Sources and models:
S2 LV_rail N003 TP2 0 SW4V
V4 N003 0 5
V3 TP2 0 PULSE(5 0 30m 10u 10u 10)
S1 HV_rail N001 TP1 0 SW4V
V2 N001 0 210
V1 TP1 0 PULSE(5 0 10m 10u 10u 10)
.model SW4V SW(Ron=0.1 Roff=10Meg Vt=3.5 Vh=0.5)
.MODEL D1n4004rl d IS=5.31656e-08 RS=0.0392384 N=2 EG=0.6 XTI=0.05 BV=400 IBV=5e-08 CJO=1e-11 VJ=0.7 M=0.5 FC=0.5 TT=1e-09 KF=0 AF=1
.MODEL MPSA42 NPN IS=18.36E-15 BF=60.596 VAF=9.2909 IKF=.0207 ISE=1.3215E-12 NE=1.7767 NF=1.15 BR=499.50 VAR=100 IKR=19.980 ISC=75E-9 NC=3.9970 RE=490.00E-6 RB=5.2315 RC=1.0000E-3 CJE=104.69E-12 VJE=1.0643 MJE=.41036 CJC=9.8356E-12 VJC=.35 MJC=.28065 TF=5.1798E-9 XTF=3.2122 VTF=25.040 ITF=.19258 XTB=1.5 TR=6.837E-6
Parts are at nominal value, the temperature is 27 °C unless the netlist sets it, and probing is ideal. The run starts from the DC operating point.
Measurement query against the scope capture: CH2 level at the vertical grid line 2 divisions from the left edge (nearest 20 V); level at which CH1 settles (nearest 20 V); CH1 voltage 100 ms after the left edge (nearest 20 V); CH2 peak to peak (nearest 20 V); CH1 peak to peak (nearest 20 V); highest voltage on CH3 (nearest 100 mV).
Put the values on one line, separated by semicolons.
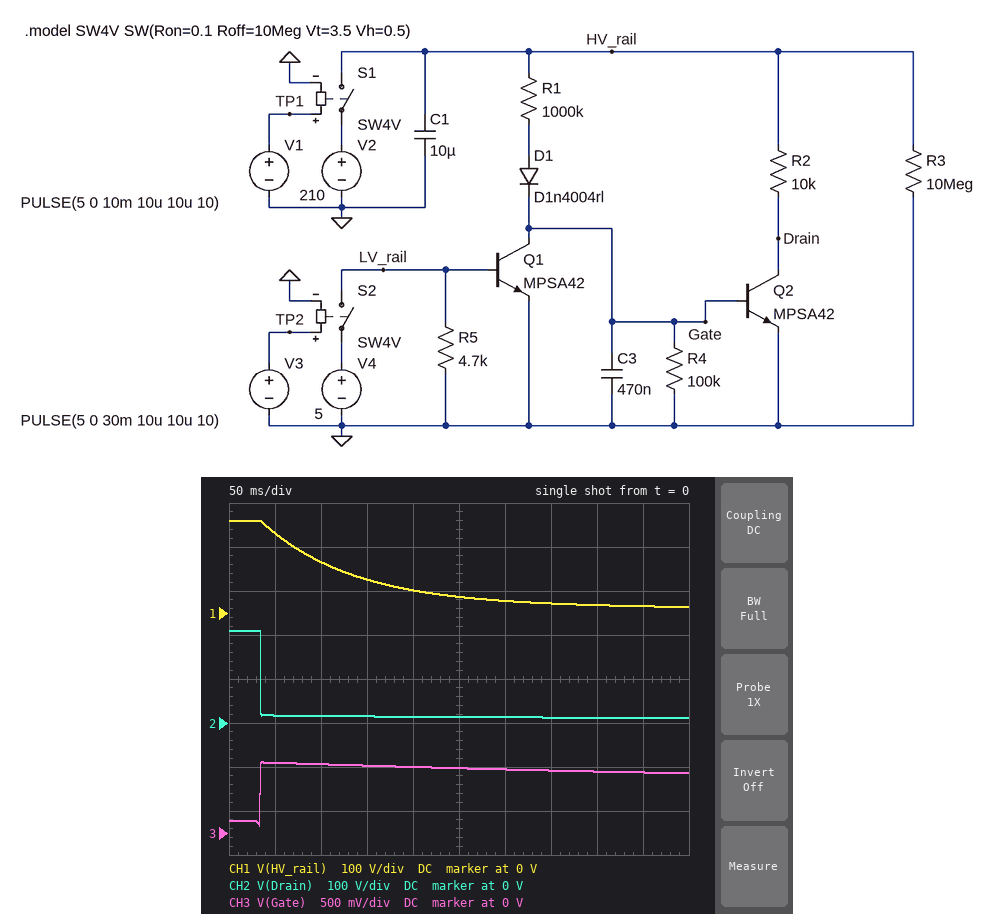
20 V; 20 V; 120 V; 200 V; 200 V; 800 mV
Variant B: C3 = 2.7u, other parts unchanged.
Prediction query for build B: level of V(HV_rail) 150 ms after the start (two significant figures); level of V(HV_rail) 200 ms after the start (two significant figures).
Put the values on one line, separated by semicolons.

80 V; 54 V
